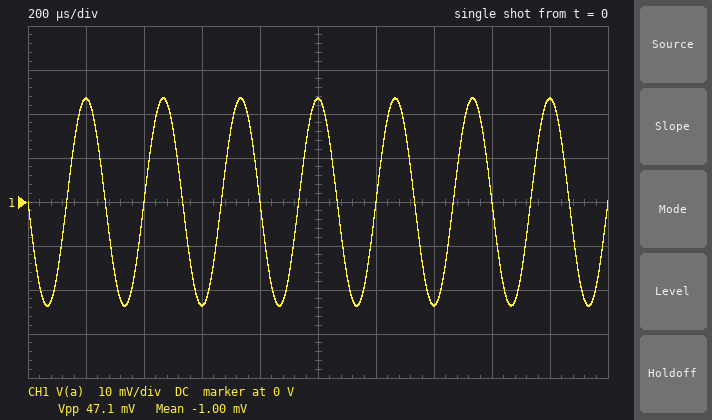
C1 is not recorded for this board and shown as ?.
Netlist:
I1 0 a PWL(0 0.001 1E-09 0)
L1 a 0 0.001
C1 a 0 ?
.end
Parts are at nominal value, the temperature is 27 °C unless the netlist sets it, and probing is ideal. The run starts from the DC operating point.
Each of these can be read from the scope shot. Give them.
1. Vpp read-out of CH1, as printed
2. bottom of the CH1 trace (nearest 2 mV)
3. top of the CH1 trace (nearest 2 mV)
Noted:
47.1 mV
-24 mV
24 mV
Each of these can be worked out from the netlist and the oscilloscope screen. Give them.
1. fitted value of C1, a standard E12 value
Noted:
1.8 µF
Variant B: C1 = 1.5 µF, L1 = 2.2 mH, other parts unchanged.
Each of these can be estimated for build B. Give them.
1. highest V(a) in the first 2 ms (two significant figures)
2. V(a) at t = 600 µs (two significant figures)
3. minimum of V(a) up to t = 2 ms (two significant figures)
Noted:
38 mV
33 mV
-38 mV
